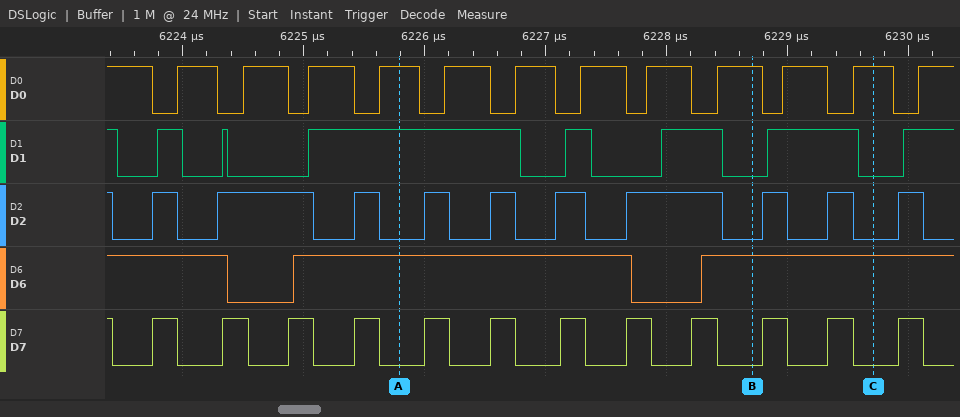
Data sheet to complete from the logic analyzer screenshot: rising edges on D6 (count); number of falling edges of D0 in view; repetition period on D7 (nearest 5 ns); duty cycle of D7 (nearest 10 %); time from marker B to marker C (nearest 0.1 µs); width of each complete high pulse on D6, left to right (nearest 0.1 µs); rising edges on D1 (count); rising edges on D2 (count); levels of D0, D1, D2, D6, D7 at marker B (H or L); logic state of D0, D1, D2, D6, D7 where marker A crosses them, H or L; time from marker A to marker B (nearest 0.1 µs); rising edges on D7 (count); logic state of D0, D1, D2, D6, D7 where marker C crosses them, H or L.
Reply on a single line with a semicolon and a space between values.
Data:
2; 12; 560 ns; 40 %; 1 µs; 2.8 µs; 7; 10; D0=H, D1=L, D2=L, D6=H, D7=L; D0=H, D1=H, D2=L, D6=H, D7=L; 2.9 µs; 12; D0=H, D1=L, D2=L, D6=H, D7=L
